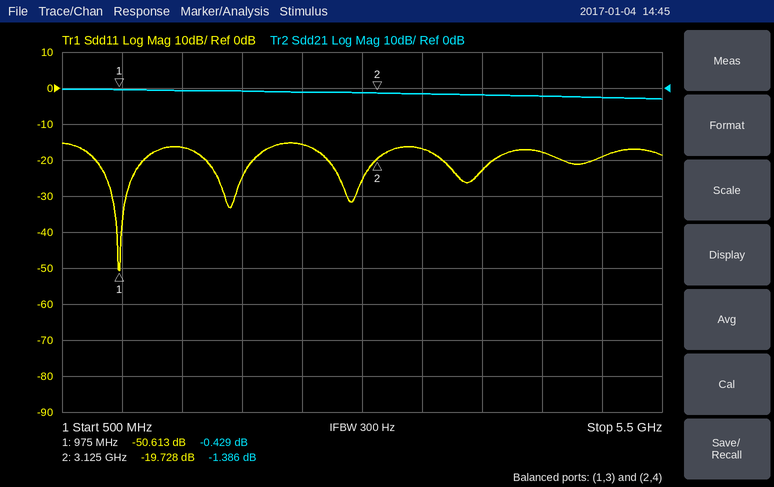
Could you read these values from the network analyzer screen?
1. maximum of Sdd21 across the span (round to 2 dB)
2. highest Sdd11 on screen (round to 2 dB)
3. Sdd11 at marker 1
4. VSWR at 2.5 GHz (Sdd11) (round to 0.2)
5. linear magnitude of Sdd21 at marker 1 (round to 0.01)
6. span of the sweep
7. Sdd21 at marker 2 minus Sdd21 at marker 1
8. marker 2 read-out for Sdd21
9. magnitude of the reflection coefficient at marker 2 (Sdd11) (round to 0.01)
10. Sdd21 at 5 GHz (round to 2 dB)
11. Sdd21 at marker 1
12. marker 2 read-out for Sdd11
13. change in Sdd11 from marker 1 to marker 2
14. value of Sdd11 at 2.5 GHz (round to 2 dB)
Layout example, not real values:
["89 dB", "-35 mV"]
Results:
["0 dB", "-16 dB", "-50.613 dB", "1.4", "0.95", "5 GHz", "-0.957 dB", "-1.386 dB", "0.10", "-2 dB", "-0.429 dB", "-19.728 dB", "30.885 dB", "-16 dB"]
